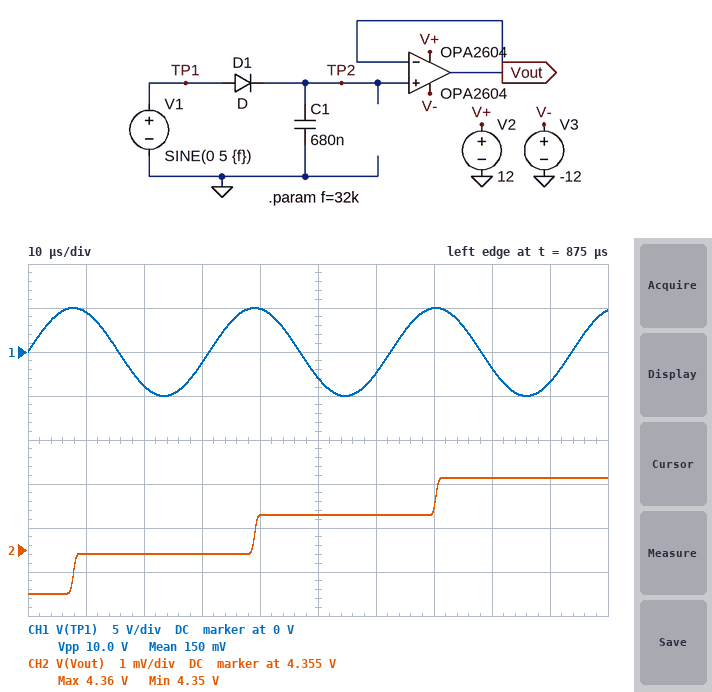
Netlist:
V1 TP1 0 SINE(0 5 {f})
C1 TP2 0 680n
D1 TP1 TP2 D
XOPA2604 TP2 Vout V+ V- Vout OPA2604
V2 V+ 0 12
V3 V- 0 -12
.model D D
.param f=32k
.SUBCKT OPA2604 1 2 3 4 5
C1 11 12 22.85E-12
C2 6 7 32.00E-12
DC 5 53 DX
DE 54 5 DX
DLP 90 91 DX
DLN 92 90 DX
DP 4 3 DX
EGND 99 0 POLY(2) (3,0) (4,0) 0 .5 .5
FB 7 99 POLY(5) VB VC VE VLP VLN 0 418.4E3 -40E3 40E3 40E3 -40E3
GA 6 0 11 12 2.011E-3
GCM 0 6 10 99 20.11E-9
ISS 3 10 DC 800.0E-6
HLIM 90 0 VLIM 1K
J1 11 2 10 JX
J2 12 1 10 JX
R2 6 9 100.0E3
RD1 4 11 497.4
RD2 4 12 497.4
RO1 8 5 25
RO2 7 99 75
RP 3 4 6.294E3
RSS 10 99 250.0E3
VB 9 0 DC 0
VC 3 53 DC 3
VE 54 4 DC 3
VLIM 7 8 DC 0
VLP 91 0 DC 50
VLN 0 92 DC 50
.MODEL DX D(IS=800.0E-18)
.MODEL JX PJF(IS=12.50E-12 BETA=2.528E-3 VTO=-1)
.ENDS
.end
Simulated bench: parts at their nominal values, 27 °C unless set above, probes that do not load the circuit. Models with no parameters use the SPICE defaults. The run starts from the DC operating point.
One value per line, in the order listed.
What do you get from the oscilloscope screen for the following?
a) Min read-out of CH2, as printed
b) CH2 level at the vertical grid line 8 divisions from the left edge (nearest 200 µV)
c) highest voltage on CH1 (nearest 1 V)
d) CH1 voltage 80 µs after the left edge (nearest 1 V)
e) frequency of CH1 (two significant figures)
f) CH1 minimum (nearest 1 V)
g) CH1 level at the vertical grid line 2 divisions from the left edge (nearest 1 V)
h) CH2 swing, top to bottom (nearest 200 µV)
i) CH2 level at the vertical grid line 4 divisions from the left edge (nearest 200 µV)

4.35 V
4.3566 V
5 V
-2 V
32 kHz
-5 V
-4 V
2.6 mV
4.3558 V
